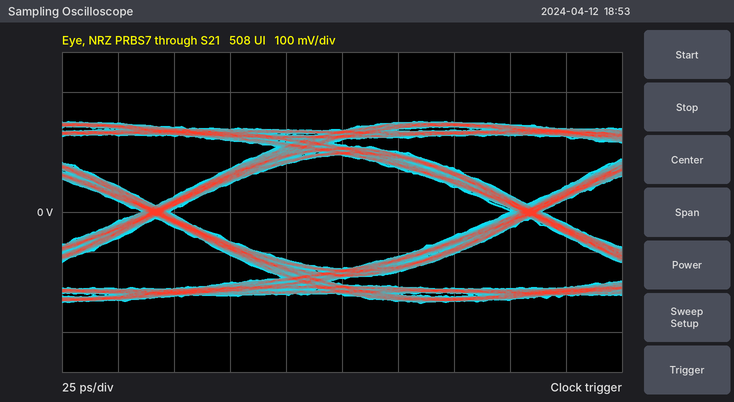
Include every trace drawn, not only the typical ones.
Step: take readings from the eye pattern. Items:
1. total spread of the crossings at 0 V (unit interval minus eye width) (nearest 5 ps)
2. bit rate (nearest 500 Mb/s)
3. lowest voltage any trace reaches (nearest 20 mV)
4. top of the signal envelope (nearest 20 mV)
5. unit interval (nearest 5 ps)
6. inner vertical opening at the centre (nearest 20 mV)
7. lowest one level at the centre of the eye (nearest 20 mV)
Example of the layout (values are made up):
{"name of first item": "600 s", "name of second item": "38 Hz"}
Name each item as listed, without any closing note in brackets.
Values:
{"total spread of the crossings at 0 V (unit interval minus eye width)": "15 ps", "bit rate": "6.0 Gb/s", "lowest voltage any trace reaches": "-220 mV", "top of the signal envelope": "220 mV", "unit interval": "165 ps", "inner vertical opening at the centre": "280 mV", "lowest one level at the centre of the eye": "140 mV"}
